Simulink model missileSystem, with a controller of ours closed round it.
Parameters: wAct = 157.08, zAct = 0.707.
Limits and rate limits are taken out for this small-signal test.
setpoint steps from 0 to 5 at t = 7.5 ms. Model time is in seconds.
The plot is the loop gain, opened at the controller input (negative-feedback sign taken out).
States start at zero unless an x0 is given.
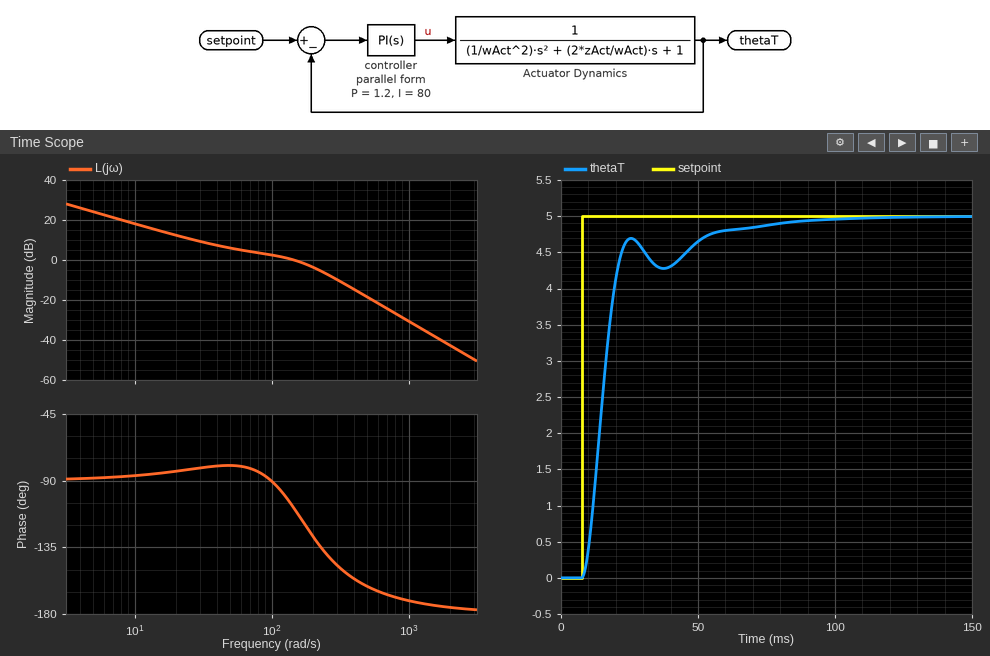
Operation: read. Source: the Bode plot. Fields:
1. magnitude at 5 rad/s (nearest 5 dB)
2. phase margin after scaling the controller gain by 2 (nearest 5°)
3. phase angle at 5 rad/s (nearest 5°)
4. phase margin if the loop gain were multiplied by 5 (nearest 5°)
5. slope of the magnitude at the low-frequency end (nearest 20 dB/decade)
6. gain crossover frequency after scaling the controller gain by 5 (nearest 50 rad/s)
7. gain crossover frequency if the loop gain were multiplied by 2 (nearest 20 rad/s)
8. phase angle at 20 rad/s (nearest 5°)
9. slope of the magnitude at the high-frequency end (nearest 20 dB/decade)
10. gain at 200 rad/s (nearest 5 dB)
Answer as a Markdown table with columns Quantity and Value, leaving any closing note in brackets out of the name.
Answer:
| Quantity | Value |
|---|---|
| magnitude at 5 rad/s | 25 dB |
| phase margin after scaling the controller gain by 2 | 45° |
| phase angle at 5 rad/s | -90° |
| phase margin if the loop gain were multiplied by 5 | 25° |
| slope of the magnitude at the low-frequency end | -20 dB/decade |
| gain crossover frequency after scaling the controller gain by 5 | 400 rad/s |
| gain crossover frequency if the loop gain were multiplied by 2 | 240 rad/s |
| phase angle at 20 rad/s | -85° |
| slope of the magnitude at the high-frequency end | -40 dB/decade |
| gain at 200 rad/s | -5 dB |
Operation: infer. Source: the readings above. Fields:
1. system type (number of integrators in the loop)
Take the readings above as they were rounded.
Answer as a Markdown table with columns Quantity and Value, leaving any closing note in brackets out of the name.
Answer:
| Quantity | Value |
|---|---|
| system type | 1 |
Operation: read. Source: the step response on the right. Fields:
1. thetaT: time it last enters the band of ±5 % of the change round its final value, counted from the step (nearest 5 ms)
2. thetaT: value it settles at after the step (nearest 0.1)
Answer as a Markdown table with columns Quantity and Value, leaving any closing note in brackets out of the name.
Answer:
| Quantity | Value |
|---|---|
| thetaT: time it last enters the band of ±5 % of the change round its final value, counted from the step | 45 ms |
| thetaT: value it settles at after the step | 5.0 |
